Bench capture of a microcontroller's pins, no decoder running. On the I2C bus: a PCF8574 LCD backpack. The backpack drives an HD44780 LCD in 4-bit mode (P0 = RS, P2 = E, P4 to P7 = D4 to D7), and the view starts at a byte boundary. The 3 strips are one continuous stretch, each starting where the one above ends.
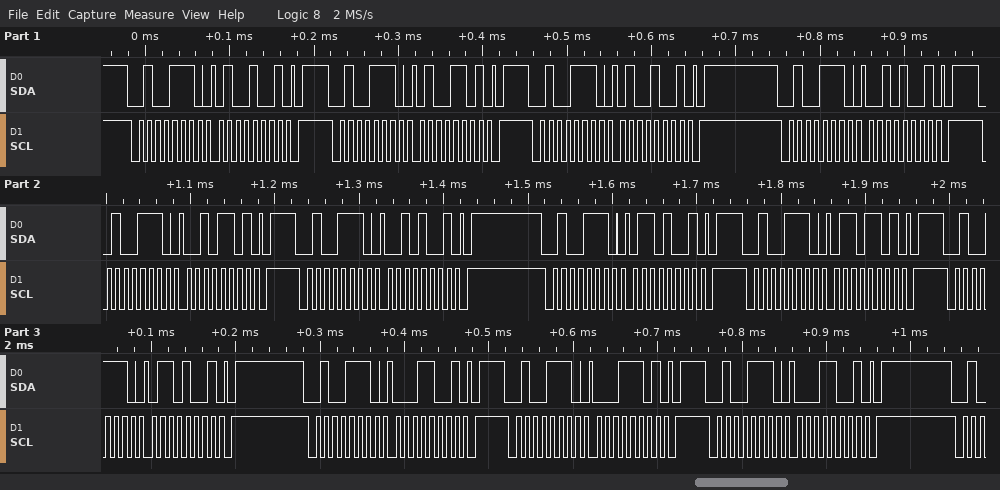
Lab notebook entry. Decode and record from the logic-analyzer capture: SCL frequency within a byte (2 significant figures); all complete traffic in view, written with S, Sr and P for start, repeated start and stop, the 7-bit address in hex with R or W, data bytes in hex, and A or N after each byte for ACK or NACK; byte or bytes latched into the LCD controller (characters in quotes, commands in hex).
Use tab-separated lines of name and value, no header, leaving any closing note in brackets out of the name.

SCL frequency within a byte	100 kHz
all complete traffic in view, written with S, Sr and P for start, repeated start and stop, the 7-bit address in hex with R or W, data bytes in hex, and A or N after each byte for ACK or NACK	S 27W A 49 A P S 27W A 4D A P S 27W A 49 A P S 27W A 29 A P S 27W A 2D A P S 27W A 29 A P S 27W A 69 A P S 27W A 6D A P S 27W A 69 A P S 27W A 19 A P S 27W A 1D A P S 27W A 19 A P
byte or bytes latched into the LCD controller	'B' 'a'
